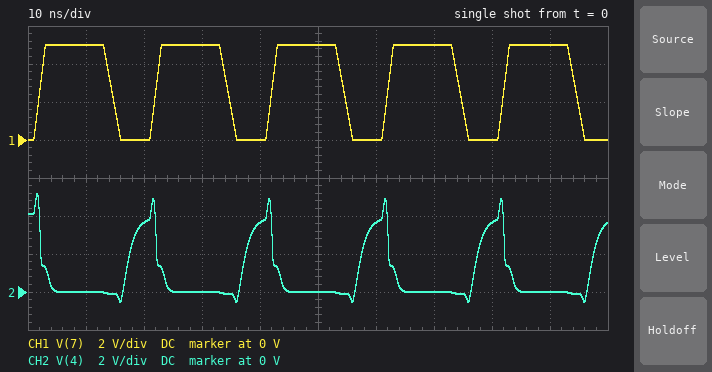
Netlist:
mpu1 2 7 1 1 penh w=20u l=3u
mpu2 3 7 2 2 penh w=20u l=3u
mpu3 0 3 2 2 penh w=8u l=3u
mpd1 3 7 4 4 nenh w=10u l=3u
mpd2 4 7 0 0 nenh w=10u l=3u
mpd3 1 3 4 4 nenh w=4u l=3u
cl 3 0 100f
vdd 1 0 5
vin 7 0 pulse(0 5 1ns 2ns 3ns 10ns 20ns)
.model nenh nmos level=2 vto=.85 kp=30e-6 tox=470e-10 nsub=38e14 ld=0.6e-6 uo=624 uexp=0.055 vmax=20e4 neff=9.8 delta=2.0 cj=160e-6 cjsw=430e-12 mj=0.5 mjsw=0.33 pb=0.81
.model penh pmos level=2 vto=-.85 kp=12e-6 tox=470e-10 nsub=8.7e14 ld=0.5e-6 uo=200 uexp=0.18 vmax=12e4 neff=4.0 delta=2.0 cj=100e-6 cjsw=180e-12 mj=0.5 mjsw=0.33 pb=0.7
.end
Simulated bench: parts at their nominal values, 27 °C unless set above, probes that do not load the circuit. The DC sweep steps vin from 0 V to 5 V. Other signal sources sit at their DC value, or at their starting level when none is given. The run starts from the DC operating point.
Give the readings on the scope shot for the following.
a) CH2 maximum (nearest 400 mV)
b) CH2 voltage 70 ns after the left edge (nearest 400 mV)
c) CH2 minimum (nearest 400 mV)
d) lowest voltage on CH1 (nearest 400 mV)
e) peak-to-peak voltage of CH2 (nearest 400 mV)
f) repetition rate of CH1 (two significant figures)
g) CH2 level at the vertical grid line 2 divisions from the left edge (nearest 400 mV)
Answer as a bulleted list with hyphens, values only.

- 5.2 V
- 0 V
- -400 mV
- 0 V
- 5.6 V
- 50 MHz
- 3.6 V
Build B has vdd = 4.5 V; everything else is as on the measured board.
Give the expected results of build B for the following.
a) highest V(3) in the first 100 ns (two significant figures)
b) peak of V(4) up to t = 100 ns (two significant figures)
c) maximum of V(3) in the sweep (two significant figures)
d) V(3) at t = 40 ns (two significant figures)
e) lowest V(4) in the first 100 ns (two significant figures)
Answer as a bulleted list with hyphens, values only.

- 4.9 V
- 4.7 V
- 4.5 V
- 4.3 V
- -550 mV
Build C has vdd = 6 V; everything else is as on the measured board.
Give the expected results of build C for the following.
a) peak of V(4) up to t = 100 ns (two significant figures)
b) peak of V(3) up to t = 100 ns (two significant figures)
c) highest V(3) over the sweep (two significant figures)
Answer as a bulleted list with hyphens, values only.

- 6.2 V
- 6.4 V
- 6.0 V
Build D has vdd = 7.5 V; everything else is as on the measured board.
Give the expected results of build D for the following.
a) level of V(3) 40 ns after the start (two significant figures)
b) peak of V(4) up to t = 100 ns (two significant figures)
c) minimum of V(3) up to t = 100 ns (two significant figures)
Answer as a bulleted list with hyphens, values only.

- 7.5 V
- 7.7 V
- -49 mV
